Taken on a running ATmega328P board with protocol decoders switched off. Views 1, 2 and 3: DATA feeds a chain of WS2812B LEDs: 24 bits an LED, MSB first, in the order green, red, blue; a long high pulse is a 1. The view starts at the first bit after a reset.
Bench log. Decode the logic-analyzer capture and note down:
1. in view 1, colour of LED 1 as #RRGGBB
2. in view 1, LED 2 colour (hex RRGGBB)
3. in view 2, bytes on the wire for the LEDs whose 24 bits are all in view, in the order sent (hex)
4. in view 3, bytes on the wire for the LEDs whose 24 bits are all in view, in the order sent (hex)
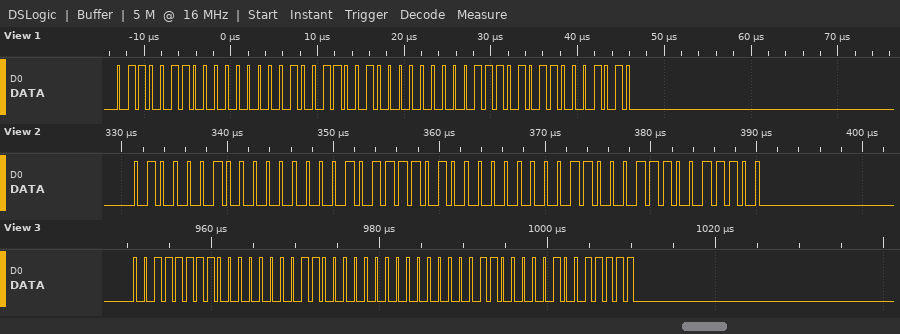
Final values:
#006699
#75008A
42 00 BD 00 63 9C
3F 00 C0 00 60 9F
